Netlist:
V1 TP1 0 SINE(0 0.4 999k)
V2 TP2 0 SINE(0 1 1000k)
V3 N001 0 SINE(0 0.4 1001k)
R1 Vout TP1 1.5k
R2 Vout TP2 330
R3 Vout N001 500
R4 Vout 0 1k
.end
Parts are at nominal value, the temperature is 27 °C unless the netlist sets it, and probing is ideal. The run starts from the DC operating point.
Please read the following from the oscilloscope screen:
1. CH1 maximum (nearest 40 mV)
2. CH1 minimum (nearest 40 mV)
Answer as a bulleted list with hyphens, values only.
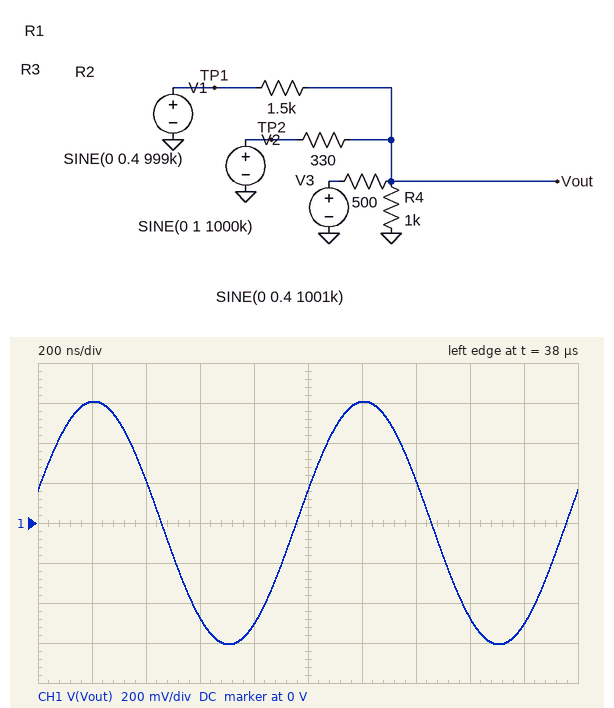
- 600 mV
- -600 mV
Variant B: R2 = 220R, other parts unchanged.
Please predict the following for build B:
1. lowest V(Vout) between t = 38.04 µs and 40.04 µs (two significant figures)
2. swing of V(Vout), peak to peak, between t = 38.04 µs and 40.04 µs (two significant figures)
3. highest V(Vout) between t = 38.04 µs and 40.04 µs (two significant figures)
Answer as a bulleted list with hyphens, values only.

- -680 mV
- 1.4 V
- 680 mV
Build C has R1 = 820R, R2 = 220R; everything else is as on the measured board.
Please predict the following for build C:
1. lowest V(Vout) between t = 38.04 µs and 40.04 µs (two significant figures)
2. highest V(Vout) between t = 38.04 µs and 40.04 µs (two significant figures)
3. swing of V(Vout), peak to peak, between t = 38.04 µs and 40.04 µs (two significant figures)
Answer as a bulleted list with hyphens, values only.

- -660 mV
- 660 mV
- 1.3 V
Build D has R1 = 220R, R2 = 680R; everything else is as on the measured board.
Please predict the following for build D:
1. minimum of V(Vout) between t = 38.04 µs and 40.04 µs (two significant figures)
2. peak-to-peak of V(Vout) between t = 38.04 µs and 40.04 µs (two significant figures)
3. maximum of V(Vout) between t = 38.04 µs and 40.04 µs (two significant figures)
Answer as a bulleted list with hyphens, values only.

- -450 mV
- 890 mV
- 450 mV
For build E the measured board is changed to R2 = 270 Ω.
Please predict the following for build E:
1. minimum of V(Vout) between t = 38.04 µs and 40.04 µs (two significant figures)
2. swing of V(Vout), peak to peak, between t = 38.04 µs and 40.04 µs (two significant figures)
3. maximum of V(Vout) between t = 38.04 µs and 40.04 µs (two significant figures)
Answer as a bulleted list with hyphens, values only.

- -640 mV
- 1.3 V
- 640 mV
